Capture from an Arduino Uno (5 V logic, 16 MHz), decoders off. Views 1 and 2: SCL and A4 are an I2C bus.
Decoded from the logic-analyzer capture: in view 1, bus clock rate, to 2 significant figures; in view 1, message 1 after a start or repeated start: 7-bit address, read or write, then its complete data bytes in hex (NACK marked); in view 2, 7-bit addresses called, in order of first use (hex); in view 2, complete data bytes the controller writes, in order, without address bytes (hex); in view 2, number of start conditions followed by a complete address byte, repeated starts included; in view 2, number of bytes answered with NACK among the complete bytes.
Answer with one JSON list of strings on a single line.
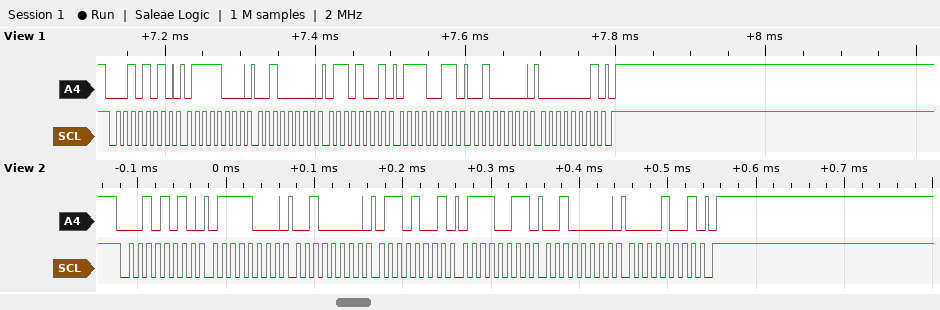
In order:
["100 kHz", "0x15 write: 78 20 69 73 20 01", "0x15", "78 20 69 73 20 09", "1", "0"]
